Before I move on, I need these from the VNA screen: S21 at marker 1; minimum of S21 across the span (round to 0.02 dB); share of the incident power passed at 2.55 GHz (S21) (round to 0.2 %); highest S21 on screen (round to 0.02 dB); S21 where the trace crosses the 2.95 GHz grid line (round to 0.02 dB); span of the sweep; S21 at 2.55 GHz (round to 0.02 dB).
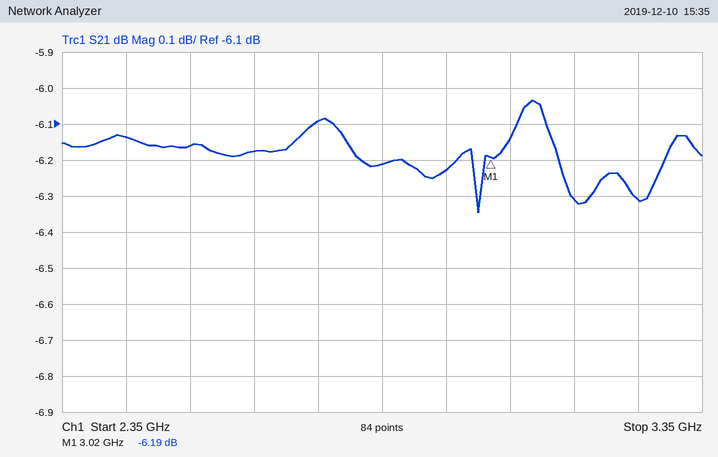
-6.19 dB
-6.34 dB
24.2 %
-6.04 dB
-6.22 dB
1 GHz
-6.16 dB
